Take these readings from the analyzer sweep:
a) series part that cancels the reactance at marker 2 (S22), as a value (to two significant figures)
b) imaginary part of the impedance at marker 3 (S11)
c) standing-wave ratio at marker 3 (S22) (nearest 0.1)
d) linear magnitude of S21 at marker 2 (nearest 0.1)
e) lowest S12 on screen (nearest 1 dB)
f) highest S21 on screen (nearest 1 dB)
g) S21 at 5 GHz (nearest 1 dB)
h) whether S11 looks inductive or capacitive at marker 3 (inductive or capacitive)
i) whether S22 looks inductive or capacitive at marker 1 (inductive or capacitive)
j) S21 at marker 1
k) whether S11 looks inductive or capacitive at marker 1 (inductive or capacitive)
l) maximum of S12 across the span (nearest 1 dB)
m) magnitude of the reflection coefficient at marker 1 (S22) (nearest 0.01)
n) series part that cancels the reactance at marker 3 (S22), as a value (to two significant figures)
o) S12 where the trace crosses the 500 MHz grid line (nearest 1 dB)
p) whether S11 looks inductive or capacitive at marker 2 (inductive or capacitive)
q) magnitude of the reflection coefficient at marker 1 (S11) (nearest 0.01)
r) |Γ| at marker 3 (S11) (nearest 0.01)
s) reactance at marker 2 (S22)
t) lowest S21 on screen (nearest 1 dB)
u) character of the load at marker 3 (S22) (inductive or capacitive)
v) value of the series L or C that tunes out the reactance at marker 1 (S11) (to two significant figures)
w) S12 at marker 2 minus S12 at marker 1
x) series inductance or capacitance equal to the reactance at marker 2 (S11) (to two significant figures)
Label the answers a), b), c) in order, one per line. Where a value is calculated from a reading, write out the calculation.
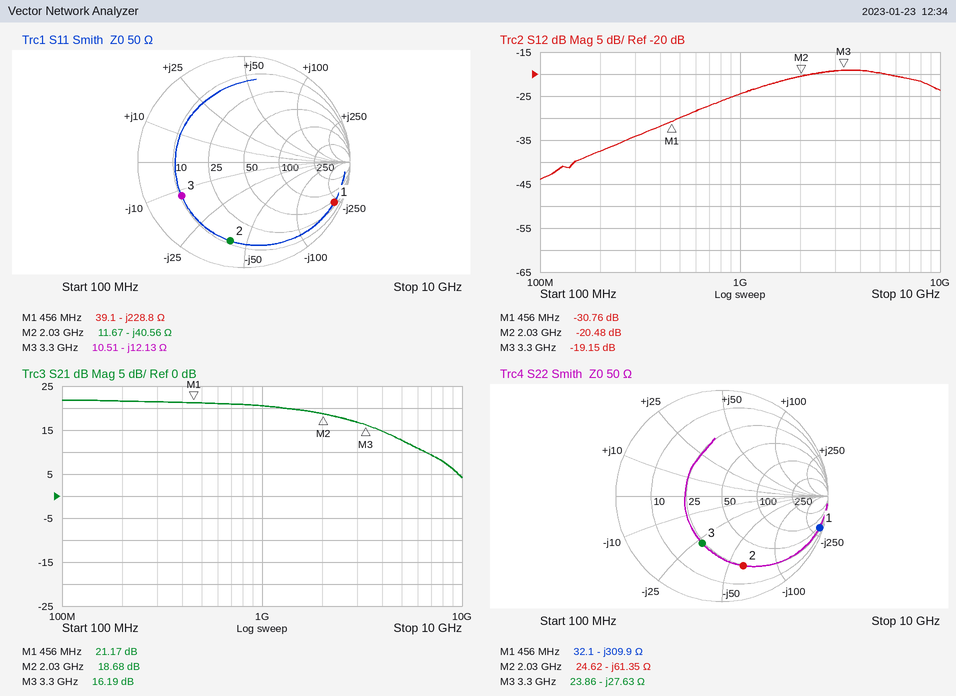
a) L = 61.35 Ω/(2π × 2.03 GHz) ≈ 4.8 nH
b) -12.13 Ω
c) 2.9
d) 10^(18.68/20) ≈ 8.6
e) -44 dB
f) 22 dB
g) 13 dB
h) capacitive
i) capacitive
j) 21.17 dB
k) capacitive
l) -19 dB
m) 0.97
n) L = 27.63 Ω/(2π × 3.3 GHz) ≈ 1.3 nH
o) -30 dB
p) capacitive
q) 0.93
r) 0.67
s) -61.35 Ω
t) 4 dB
u) capacitive
v) L = 228.8 Ω/(2π × 456 MHz) ≈ 80 nH
w) -20.48 − (-30.76) = 10.28 dB
x) C = 1/(2π × 2.03 GHz × 40.56 Ω) ≈ 1.9 pF
